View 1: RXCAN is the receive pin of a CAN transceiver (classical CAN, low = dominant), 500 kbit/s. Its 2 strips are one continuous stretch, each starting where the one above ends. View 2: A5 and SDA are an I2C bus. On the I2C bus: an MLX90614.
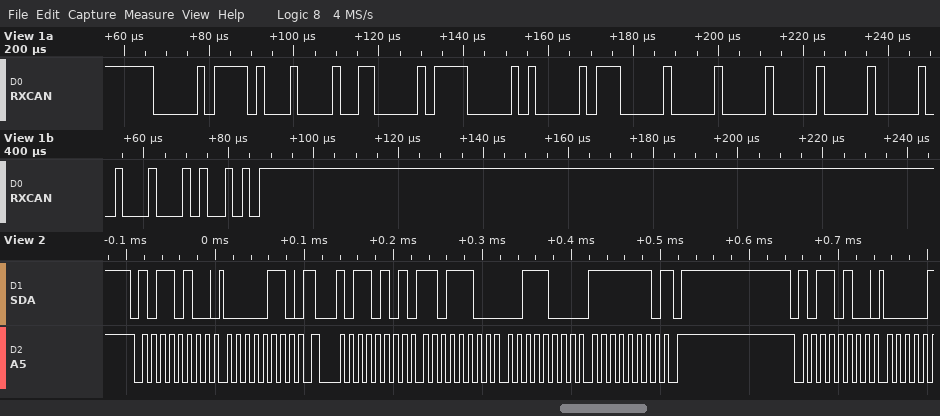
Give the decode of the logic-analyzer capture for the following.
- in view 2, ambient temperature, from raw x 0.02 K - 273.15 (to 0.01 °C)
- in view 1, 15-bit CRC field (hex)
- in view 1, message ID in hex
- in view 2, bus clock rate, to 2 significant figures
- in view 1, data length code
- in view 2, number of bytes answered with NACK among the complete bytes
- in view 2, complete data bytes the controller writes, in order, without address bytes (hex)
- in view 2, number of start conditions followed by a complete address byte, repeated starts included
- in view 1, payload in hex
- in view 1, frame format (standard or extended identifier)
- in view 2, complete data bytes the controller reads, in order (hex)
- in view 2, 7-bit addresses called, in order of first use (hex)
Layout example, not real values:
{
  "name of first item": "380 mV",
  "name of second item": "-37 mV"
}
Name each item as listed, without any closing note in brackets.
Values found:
{
  "in view 2, ambient temperature, from raw x 0.02 K - 273.15": "17.97 °C",
  "in view 1, 15-bit CRC field": "0x4452",
  "in view 1, message ID in hex": "0x03D",
  "in view 2, bus clock rate, to 2 significant figures": "100 kHz",
  "in view 1, data length code": "8",
  "in view 2, number of bytes answered with NACK among the complete bytes": "1",
  "in view 2, complete data bytes the controller writes, in order, without address bytes": "06",
  "in view 2, number of start conditions followed by a complete address byte, repeated starts included": "3",
  "in view 1, payload in hex": "4C 0F 02 07 00 00 00 00",
  "in view 1, frame format": "standard",
  "in view 2, complete data bytes the controller reads, in order": "DC 38 FE",
  "in view 2, 7-bit addresses called, in order of first use": "0x5A"
}
